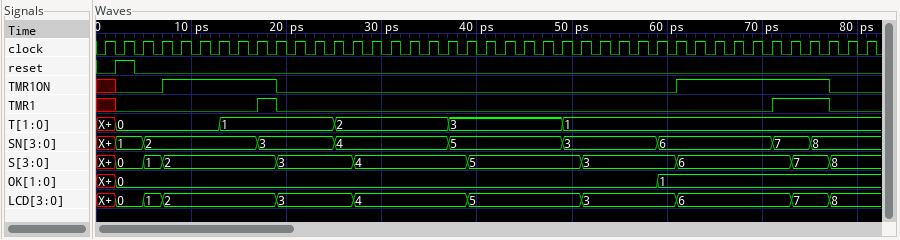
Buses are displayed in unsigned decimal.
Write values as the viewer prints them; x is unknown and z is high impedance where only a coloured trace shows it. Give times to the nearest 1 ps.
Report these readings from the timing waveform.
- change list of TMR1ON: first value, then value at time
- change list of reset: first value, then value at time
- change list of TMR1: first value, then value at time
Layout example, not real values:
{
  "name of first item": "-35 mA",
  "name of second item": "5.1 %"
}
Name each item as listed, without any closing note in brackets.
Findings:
{
  "change list of TMR1ON: first value, then value at time": "x, 0 at 2 ps, 1 at 7 ps, 0 at 19 ps, 1 at 61 ps, 0 at 77 ps",
  "change list of reset: first value, then value at time": "0, 1 at 2 ps, 0 at 4 ps",
  "change list of TMR1: first value, then value at time": "x, 0 at 2 ps, 1 at 17 ps, 0 at 19 ps, 1 at 71 ps, 0 at 77 ps"
}
